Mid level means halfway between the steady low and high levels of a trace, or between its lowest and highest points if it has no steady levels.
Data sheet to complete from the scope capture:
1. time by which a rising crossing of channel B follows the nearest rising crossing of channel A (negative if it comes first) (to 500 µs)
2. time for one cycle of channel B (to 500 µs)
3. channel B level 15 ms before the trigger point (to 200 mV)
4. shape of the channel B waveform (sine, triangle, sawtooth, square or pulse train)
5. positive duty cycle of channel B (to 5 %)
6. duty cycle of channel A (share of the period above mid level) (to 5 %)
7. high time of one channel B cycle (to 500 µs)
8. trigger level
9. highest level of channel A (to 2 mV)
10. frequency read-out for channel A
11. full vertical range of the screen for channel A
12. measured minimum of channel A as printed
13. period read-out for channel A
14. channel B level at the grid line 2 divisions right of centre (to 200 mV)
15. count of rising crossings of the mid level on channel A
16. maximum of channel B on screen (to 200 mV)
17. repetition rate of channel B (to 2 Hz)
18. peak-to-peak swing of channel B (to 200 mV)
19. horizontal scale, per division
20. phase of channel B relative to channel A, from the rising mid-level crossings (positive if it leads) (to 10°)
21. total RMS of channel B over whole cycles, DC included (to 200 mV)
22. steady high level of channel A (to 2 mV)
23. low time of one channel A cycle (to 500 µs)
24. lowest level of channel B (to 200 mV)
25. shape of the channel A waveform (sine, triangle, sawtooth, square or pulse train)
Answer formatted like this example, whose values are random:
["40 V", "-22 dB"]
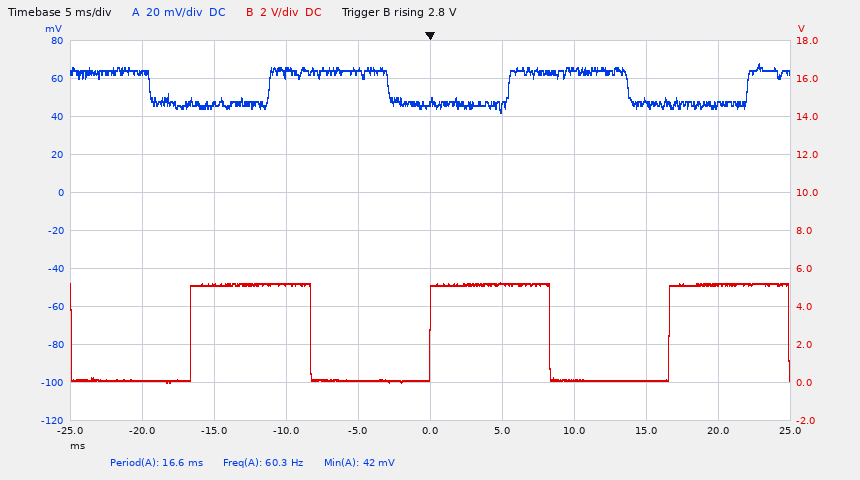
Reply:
["-5.5 ms", "16.5 ms", "5.2 V", "square", "50 %", "50 %", "8.5 ms", "2.8 V", "68 mV", "60.3 Hz", "200 mV", "42 mV", "16.6 ms", "200 mV", "3", "5.2 V", "60 Hz", "5.2 V", "5 ms", "+120°", "3.6 V", "64 mV", "8.5 ms", "0.0 V", "square"]
